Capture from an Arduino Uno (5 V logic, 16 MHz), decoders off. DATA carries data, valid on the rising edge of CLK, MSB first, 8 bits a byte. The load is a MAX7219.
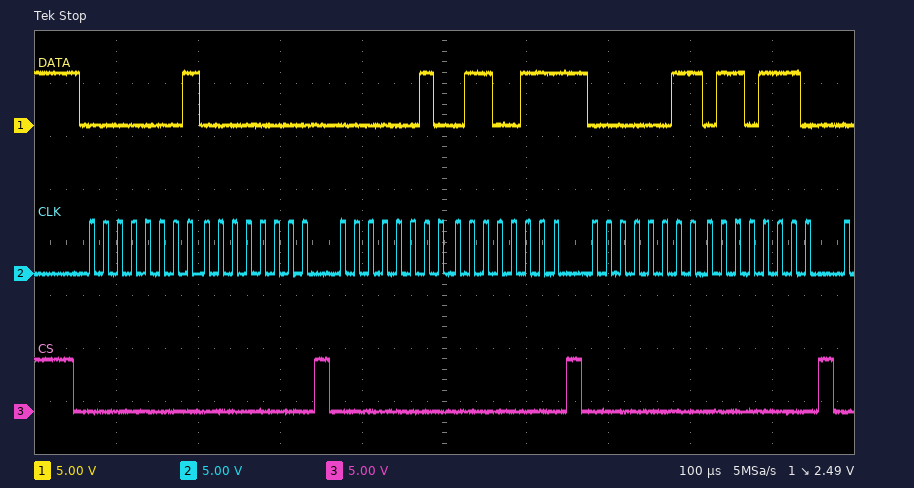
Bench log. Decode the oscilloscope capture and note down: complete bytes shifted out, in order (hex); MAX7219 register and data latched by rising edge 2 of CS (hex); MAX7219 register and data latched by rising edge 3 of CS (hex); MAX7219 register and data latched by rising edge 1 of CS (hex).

01 00 02 67 03 6E
register 0x2, data 0x67
register 0x3, data 0x6E
register 0x1, data 0x00
